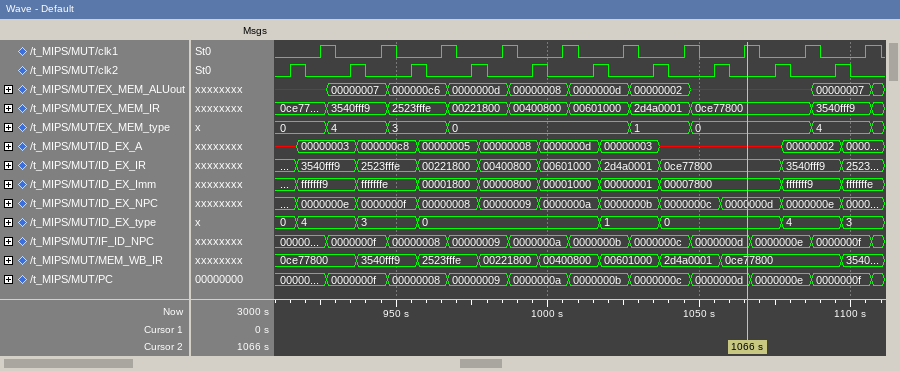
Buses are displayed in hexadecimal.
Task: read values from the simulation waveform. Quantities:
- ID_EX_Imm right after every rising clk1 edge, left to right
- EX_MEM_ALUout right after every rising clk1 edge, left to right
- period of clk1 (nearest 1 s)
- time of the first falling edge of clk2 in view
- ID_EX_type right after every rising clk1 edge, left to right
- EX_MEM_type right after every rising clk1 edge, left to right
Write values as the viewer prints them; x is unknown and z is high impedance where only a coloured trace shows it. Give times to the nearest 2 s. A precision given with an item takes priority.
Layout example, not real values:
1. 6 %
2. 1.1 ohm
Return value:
1. fffffff9, fffffffe, 00001800, 00000800, 00001000, 00000001, 00007800, 00007800, fffffff9, fffffffe
2. x, 00000007, 000000c6, 0000000d, 00000008, 0000000d, 00000002, x, x, 00000007
3. 20 s
4. 920 s
5. 4, 3, 0, 0, 0, 1, 0, 0, 4, 3
6. 0, 4, 3, 0, 0, 0, 1, 0, 0, 4
